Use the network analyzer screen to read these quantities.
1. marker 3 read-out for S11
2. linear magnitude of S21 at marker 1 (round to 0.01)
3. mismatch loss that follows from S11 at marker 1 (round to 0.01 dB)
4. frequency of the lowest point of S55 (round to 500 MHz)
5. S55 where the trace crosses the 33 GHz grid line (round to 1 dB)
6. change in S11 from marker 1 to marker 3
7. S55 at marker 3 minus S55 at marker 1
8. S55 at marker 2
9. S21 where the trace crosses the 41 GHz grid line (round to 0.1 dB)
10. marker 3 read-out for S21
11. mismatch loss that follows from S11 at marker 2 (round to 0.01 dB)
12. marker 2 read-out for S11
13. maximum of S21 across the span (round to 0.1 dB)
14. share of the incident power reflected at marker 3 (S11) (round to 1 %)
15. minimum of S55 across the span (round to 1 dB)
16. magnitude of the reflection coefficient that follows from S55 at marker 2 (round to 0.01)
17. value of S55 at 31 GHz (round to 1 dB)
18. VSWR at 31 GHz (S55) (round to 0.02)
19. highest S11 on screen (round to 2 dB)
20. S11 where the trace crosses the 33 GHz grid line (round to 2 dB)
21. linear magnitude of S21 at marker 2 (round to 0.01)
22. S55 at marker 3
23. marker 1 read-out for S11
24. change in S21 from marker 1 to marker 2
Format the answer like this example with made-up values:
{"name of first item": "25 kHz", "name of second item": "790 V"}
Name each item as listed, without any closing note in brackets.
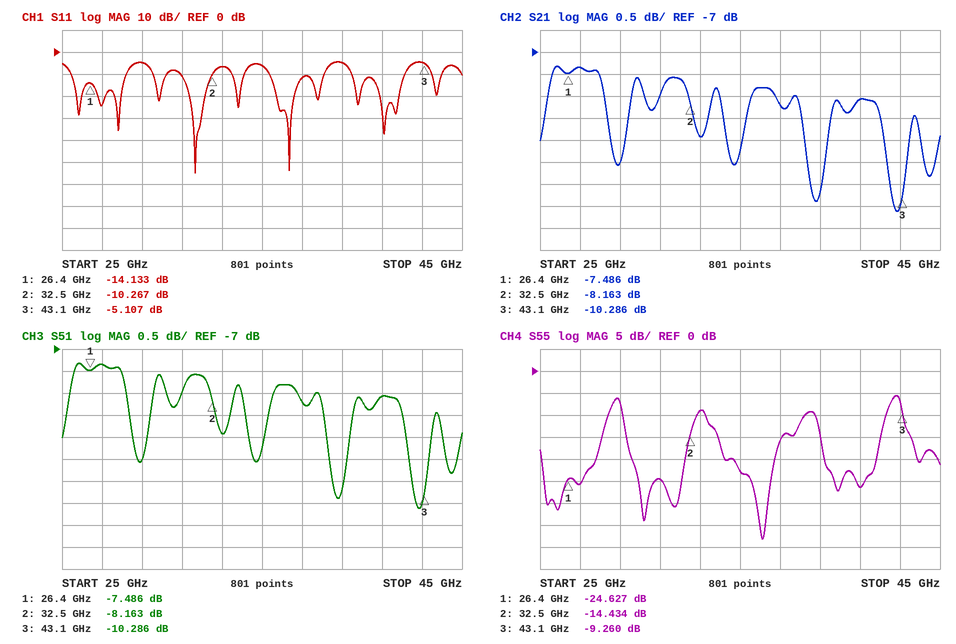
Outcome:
{"marker 3 read-out for S11": "-5.107 dB", "linear magnitude of S21 at marker 1": "0.42", "mismatch loss that follows from S11 at marker 1": "0.17 dB", "frequency of the lowest point of S55": "36.0 GHz", "S55 where the trace crosses the 33 GHz grid line": "-9 dB", "change in S11 from marker 1 to marker 3": "9.026 dB", "S55 at marker 3 minus S55 at marker 1": "15.367 dB", "S55 at marker 2": "-14.434 dB", "S21 where the trace crosses the 41 GHz grid line": "-8.1 dB", "marker 3 read-out for S21": "-10.286 dB", "mismatch loss that follows from S11 at marker 2": "0.43 dB", "marker 2 read-out for S11": "-10.267 dB", "maximum of S21 across the span": "-7.3 dB", "share of the incident power reflected at marker 3 (S11)": "31 %", "minimum of S55 across the span": "-38 dB", "magnitude of the reflection coefficient that follows from S55 at marker 2": "0.19", "value of S55 at 31 GHz": "-25 dB", "VSWR at 31 GHz (S55)": "1.12", "highest S11 on screen": "-4 dB", "S11 where the trace crosses the 33 GHz grid line": "-6 dB", "linear magnitude of S21 at marker 2": "0.39", "S55 at marker 3": "-9.260 dB", "marker 1 read-out for S11": "-14.133 dB", "change in S21 from marker 1 to marker 2": "-0.677 dB"}
